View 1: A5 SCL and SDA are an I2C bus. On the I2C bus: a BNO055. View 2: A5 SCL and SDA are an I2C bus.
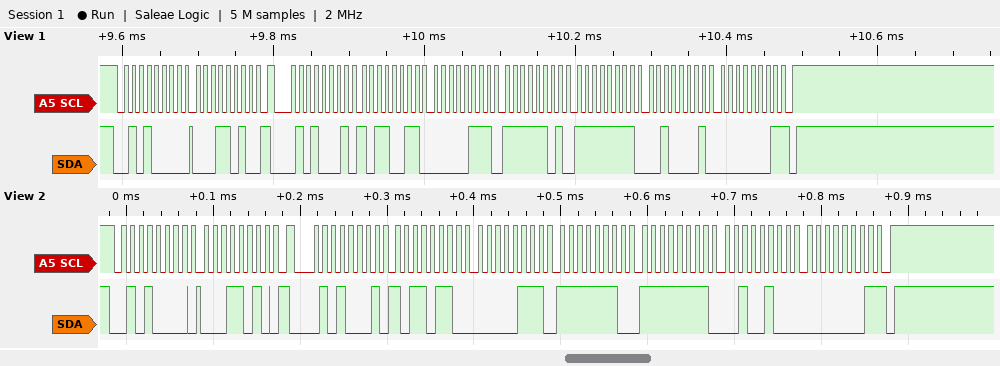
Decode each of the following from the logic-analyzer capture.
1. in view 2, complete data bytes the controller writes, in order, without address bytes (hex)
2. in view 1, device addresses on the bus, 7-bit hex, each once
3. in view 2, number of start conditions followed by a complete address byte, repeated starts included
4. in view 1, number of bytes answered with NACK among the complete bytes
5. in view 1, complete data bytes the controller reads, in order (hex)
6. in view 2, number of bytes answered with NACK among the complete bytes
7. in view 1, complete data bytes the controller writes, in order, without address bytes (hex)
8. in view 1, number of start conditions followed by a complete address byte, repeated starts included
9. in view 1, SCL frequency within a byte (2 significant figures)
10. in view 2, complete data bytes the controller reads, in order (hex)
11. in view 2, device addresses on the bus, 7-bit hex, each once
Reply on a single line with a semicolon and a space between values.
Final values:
1A; 0x28; 2; 1; B3 07 FD FF 21 01; 1; 1A; 2; 100 kHz; B6 07 FE FF 24 01; 0x28
